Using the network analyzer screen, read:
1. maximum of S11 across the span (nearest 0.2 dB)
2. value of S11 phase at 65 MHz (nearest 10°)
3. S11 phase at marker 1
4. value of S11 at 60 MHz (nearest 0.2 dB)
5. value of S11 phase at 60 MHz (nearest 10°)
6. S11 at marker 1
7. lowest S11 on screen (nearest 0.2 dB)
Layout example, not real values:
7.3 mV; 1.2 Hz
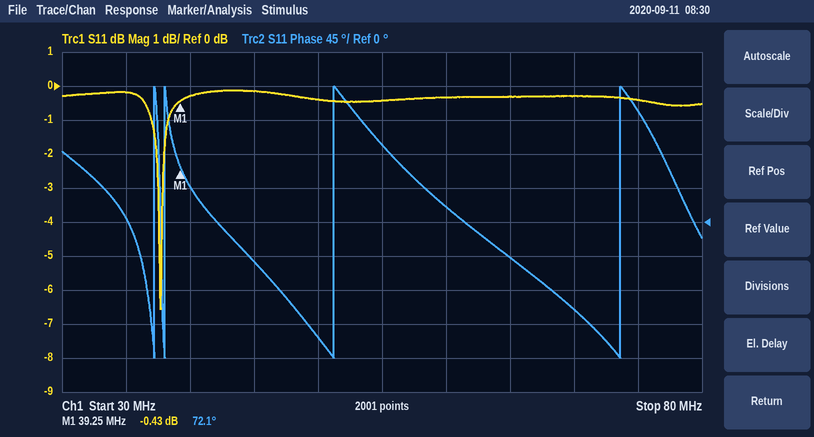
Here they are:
-0.2 dB; -50°; 72.1°; -0.4 dB; 20°; -0.43 dB; -6.6 dB
